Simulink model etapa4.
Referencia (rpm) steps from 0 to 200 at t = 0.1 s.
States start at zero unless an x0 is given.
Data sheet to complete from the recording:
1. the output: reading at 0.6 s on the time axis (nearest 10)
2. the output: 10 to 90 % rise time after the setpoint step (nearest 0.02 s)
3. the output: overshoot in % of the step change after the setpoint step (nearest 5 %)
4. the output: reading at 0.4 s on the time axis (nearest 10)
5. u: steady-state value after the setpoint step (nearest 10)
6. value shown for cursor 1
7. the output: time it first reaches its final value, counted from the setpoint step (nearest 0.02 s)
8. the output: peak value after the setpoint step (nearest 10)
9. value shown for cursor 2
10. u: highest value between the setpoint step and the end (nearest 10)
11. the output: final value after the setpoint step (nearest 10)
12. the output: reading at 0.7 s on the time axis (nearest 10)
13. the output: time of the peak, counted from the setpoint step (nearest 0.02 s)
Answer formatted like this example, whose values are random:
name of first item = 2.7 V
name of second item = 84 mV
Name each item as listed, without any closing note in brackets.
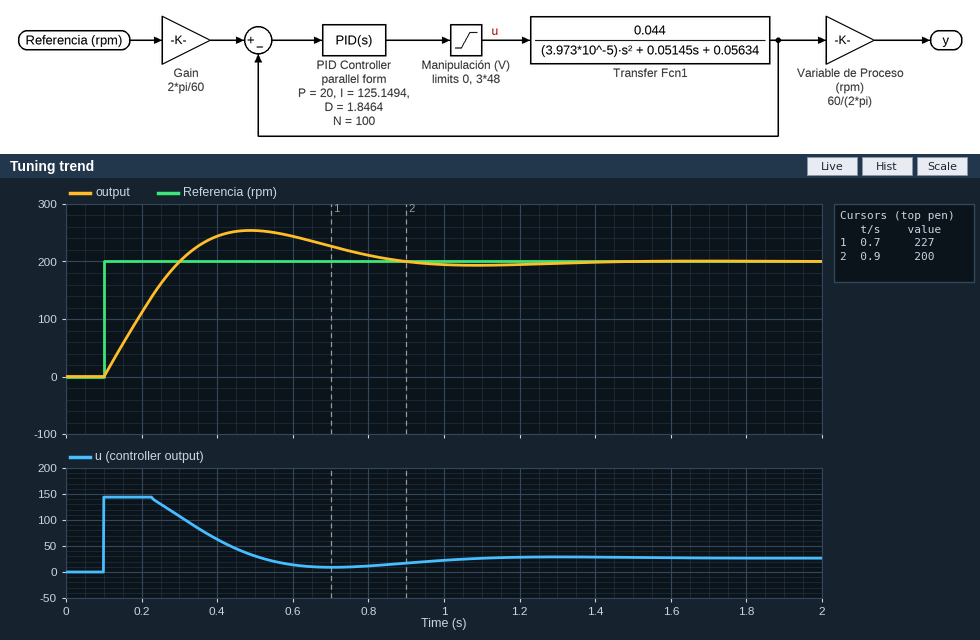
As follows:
the output: reading at 0.6 s on the time axis = 240
the output: 10 to 90 % rise time after the setpoint step = 0.16 s
the output: overshoot in % of the step change after the setpoint step = 25 %
the output: reading at 0.4 s on the time axis = 240
u: steady-state value after the setpoint step = 30
value shown for cursor 1 = 227
the output: time it first reaches its final value, counted from the setpoint step = 0.20 s
the output: peak value after the setpoint step = 250
value shown for cursor 2 = 200
u: highest value between the setpoint step and the end = 140
the output: final value after the setpoint step = 200
the output: reading at 0.7 s on the time axis = 230
the output: time of the peak, counted from the setpoint step = 0.38 s
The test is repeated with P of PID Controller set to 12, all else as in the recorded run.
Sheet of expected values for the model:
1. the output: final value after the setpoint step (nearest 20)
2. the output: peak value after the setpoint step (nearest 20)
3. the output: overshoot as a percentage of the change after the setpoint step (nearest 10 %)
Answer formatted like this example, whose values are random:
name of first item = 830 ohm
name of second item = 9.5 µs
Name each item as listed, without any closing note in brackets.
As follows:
the output: final value after the setpoint step = 200
the output: peak value after the setpoint step = 280
the output: overshoot as a percentage of the change after the setpoint step = 40 %
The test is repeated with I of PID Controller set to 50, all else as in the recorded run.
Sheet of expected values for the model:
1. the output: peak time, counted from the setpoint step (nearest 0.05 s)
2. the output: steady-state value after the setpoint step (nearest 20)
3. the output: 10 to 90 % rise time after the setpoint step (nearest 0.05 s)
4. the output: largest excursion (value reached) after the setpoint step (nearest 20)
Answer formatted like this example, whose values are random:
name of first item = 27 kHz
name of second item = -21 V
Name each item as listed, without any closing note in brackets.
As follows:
the output: peak time, counted from the setpoint step = 0.55 s
the output: steady-state value after the setpoint step = 200
the output: 10 to 90 % rise time after the setpoint step = 0.20 s
the output: largest excursion (value reached) after the setpoint step = 220
